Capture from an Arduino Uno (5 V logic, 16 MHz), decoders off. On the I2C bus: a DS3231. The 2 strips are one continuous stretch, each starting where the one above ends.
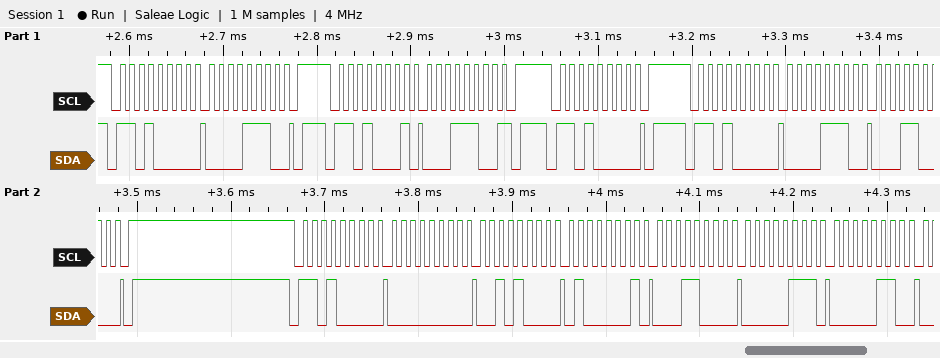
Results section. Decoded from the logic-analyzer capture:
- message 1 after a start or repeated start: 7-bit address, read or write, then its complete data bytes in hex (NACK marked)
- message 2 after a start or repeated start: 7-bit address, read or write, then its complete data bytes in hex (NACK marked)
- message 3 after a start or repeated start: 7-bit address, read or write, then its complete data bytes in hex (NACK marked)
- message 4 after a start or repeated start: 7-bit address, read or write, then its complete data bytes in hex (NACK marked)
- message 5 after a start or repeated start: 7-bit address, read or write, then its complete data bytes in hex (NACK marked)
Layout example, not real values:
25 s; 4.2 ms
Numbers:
0x68 write: 0E; 0x68 read: 1C NACK; 0x68 write; 0x68 write: 0E 18; 0x68 write: 00 28 41 18 07 06
